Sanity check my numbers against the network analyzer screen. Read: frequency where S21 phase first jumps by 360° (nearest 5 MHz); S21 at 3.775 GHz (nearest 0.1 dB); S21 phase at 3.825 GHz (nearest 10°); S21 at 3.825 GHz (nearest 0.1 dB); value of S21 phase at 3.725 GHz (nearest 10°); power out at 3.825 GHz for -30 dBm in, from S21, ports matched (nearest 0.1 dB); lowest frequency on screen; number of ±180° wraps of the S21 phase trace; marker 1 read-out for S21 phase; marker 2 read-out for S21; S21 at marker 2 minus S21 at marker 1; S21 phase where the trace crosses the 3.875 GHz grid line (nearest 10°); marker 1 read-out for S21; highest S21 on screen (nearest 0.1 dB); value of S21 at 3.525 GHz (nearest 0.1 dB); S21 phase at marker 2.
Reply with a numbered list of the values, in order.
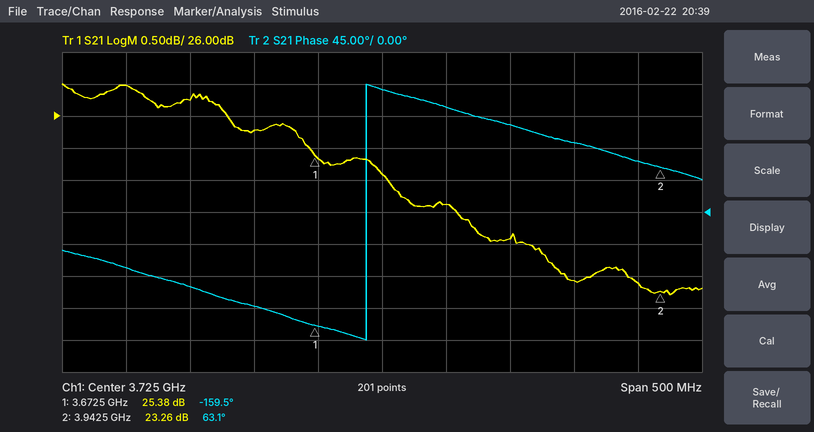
1. 3.715 GHz
2. 24.6 dB
3. 120°
4. 24.1 dB
5. 170°
6. -5.9 dBm
7. 3.475 GHz
8. 1
9. -159.5°
10. 23.26 dB
11. -2.12 dB
12. 100°
13. 25.38 dB
14. 26.5 dB
15. 26.5 dB
16. 63.1°
